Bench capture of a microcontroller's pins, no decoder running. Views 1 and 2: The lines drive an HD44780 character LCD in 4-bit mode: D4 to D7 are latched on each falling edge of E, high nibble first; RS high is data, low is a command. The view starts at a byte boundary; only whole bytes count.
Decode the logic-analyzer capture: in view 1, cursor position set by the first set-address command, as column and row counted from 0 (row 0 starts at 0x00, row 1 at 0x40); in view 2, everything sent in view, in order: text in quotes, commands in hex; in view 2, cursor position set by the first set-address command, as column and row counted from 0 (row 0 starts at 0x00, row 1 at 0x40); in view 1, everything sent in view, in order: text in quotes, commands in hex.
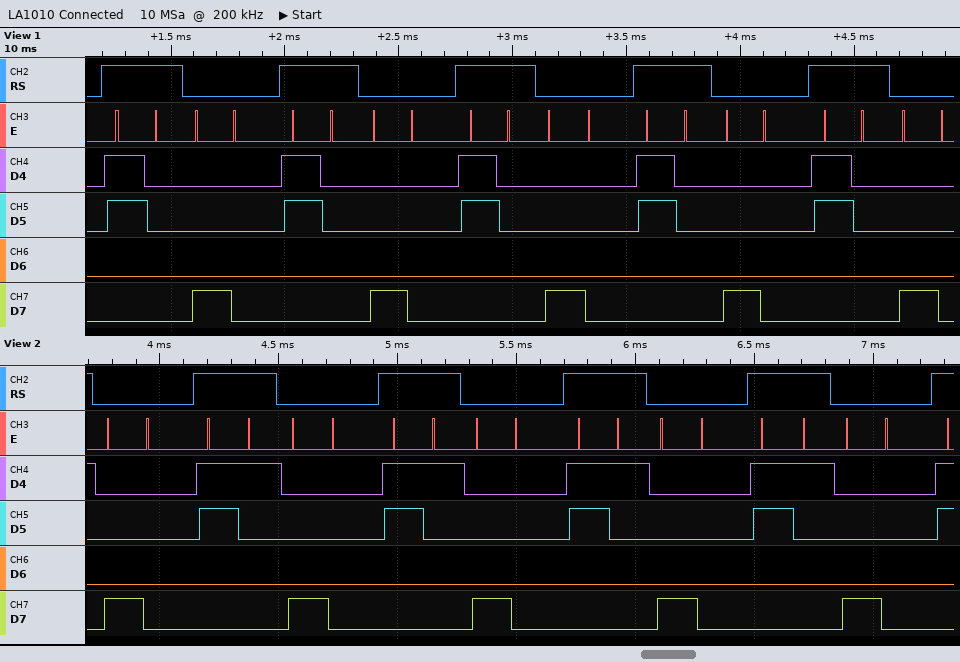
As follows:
column 0, row 0
0x80 "1" 0x80 "1" 0x80 "1" 0x80 "1" 0x80
column 0, row 0
"0" 0x80 "0" 0x80 "0" 0x80 "0" 0x80 "0" 0x80
